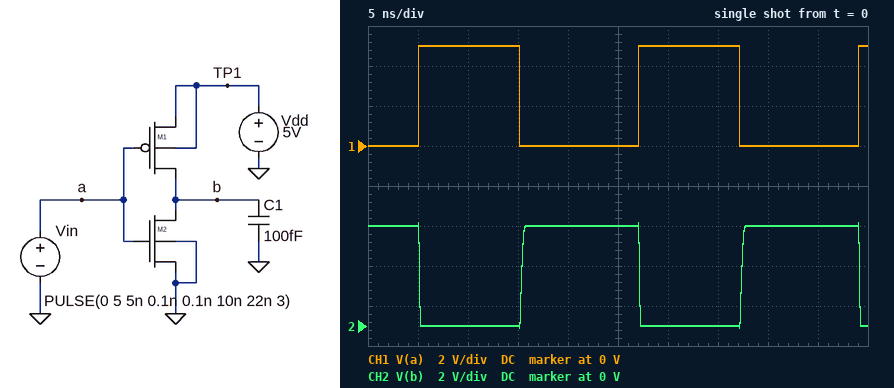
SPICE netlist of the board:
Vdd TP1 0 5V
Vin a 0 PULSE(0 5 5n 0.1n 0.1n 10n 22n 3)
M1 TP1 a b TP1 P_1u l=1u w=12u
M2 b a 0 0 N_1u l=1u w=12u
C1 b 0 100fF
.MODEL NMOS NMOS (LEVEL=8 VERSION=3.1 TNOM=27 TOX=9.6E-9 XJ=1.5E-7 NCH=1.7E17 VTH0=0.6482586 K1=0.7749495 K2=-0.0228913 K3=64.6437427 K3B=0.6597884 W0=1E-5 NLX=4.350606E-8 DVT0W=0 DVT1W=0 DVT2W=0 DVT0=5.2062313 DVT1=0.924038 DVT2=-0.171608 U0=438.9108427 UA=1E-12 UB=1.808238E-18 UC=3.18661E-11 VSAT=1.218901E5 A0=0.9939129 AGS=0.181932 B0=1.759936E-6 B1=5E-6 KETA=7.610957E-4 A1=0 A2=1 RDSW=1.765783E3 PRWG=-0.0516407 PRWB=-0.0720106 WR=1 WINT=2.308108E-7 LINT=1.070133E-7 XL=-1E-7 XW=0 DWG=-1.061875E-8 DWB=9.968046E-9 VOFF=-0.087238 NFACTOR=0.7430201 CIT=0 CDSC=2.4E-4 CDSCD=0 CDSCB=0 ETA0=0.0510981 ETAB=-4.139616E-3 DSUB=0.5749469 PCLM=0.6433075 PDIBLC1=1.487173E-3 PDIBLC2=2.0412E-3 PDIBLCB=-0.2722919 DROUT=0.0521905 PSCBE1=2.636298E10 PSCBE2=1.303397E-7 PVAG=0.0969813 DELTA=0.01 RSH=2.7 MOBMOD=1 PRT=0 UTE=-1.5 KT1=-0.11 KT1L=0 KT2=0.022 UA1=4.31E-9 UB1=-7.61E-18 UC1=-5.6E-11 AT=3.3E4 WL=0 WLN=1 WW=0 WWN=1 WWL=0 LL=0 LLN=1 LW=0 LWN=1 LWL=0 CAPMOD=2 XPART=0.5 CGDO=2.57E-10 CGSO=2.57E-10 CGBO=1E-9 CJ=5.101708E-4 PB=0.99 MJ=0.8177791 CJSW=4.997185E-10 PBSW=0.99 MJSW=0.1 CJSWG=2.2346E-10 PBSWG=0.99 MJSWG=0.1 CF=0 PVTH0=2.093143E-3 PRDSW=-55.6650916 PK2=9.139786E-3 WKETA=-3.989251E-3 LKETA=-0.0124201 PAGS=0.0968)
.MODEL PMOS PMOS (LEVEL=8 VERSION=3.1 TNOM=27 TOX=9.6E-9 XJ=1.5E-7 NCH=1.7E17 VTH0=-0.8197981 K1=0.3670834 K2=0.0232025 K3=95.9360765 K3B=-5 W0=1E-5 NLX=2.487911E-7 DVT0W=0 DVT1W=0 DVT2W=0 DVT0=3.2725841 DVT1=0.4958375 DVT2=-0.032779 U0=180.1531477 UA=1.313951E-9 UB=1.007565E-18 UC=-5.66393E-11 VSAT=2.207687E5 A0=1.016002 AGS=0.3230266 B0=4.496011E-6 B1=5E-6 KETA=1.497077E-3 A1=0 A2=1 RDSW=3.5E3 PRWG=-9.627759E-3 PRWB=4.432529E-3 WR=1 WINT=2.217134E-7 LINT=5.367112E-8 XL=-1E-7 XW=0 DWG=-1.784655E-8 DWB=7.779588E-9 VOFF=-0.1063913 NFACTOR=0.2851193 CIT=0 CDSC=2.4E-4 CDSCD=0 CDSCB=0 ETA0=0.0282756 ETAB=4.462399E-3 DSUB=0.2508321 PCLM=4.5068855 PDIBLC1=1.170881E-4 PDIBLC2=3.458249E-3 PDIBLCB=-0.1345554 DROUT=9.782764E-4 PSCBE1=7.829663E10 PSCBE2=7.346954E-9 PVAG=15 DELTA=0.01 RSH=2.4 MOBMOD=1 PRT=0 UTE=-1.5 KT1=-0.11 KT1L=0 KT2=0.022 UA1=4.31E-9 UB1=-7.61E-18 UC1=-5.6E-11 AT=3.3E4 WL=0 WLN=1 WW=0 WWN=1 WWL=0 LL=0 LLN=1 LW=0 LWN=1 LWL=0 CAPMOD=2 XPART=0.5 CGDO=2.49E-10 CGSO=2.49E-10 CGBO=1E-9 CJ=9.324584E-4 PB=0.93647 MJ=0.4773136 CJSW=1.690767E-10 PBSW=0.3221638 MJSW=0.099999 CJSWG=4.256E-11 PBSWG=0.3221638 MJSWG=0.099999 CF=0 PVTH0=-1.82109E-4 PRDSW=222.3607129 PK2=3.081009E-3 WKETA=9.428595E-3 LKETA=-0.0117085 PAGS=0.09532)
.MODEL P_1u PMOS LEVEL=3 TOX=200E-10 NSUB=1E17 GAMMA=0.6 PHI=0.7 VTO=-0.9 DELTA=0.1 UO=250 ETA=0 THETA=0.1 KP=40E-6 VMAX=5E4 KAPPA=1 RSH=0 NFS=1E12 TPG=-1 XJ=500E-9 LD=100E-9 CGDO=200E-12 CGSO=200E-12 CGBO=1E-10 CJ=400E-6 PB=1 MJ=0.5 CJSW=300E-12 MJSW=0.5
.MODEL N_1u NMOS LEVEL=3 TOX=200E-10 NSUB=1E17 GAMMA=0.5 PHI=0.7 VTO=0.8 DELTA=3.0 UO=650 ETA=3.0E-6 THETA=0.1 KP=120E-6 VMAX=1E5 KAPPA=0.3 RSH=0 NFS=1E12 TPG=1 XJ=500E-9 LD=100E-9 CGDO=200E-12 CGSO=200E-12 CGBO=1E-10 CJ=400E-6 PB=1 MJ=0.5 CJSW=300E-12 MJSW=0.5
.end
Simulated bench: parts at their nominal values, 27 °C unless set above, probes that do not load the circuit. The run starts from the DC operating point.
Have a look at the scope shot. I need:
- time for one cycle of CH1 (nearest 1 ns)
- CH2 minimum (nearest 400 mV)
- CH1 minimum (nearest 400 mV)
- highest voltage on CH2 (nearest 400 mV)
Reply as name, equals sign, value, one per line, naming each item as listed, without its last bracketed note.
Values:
time for one cycle of CH1 = 22 ns
CH2 minimum = 0 V
CH1 minimum = 0 V
highest voltage on CH2 = 5.2 V
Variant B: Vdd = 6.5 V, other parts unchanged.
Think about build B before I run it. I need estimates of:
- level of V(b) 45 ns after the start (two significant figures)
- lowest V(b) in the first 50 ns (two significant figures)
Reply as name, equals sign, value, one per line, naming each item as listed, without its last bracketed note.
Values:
level of V(b) 45 ns after the start = 6.5 V
lowest V(b) in the first 50 ns = -31 mV
